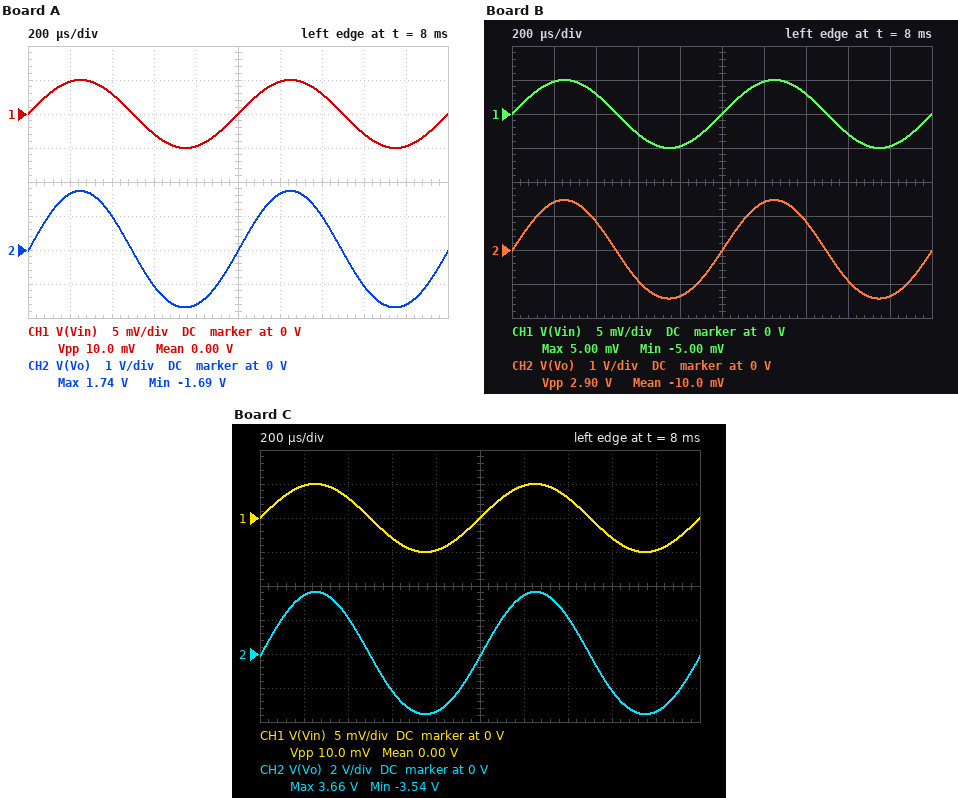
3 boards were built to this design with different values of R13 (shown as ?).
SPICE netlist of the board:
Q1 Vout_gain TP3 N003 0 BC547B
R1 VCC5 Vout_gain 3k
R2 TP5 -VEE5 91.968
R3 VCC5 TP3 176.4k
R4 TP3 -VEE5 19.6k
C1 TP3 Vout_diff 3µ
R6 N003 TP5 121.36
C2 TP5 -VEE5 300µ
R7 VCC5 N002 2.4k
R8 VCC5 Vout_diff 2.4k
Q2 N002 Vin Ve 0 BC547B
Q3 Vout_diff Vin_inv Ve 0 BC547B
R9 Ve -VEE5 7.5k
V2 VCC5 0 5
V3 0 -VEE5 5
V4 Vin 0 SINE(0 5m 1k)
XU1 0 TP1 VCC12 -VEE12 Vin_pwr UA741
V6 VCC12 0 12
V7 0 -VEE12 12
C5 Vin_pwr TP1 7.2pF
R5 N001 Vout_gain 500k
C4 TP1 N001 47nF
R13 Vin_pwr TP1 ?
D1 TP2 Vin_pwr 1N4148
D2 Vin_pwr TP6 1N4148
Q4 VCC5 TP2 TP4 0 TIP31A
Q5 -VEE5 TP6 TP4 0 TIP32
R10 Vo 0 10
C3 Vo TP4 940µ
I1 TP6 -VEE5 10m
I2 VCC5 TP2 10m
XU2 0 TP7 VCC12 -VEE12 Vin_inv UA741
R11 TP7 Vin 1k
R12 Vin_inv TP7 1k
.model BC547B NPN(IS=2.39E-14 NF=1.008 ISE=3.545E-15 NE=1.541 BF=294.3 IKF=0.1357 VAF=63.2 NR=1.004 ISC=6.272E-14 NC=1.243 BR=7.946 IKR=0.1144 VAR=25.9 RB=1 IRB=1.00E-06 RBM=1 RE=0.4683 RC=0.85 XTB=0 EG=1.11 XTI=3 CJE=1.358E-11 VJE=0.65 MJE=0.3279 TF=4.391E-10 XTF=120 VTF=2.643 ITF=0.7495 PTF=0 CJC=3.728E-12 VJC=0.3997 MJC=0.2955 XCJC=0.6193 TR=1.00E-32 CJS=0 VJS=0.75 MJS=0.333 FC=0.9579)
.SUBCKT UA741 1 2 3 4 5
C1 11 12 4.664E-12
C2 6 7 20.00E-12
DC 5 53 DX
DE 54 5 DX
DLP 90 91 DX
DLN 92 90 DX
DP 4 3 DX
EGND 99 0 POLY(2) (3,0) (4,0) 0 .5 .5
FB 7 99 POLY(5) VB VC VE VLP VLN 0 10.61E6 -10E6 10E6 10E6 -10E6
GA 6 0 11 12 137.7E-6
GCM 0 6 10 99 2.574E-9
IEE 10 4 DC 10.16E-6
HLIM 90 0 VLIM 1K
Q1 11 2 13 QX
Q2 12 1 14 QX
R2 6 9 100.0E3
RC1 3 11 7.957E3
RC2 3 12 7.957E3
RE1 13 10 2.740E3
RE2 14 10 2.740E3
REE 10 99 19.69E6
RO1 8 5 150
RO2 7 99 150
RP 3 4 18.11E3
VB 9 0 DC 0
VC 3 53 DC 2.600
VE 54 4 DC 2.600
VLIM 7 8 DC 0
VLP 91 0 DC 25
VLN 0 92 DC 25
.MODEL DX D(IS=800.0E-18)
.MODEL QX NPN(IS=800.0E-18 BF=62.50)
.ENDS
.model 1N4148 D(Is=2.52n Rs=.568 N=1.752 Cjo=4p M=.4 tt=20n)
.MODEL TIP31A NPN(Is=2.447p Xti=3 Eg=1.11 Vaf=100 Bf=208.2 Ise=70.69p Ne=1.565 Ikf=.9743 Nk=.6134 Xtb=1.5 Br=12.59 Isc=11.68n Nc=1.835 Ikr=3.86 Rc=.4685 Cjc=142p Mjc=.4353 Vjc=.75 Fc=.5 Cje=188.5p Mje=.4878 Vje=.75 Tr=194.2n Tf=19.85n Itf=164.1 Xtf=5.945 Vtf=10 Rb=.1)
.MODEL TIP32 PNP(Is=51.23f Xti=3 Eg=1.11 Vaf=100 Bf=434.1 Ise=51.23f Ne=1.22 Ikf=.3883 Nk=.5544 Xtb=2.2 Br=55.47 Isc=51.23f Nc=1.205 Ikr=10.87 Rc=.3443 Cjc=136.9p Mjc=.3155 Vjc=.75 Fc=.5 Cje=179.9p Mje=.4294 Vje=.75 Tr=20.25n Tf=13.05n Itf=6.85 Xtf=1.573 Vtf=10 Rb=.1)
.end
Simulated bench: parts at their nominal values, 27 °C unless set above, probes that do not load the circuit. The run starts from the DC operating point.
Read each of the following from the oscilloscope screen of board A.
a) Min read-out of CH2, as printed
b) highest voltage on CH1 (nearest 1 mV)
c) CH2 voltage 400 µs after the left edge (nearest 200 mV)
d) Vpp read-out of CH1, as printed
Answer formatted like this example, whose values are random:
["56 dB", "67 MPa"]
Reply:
["-1.69 V", "5 mV", "1.0 V", "10.0 mV"]
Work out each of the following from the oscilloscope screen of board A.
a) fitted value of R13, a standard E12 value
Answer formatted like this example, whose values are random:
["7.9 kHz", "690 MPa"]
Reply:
["390 kΩ"]
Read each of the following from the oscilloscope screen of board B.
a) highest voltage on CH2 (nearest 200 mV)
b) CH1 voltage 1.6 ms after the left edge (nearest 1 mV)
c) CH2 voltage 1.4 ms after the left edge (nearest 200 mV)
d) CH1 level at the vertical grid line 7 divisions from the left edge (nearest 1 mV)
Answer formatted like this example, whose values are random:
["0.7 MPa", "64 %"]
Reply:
["1.4 V", "-3 mV", "800 mV", "3 mV"]
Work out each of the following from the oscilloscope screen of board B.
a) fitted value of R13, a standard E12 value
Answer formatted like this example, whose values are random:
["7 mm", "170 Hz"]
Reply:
["330 kΩ"]
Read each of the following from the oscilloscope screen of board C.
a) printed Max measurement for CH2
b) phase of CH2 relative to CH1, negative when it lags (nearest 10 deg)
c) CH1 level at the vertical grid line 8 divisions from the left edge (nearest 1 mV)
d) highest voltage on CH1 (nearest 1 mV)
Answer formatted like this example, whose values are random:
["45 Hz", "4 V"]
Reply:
["3.66 V", "0 deg", "-3 mV", "5 mV"]
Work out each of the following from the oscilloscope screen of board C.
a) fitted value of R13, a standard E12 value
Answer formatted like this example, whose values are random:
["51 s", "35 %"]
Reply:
["820 kΩ"]
